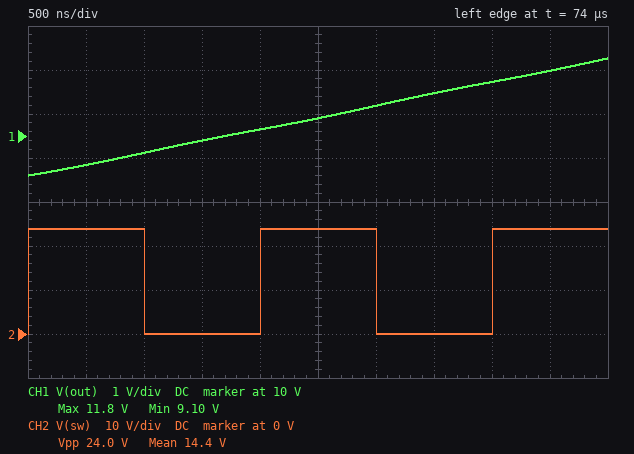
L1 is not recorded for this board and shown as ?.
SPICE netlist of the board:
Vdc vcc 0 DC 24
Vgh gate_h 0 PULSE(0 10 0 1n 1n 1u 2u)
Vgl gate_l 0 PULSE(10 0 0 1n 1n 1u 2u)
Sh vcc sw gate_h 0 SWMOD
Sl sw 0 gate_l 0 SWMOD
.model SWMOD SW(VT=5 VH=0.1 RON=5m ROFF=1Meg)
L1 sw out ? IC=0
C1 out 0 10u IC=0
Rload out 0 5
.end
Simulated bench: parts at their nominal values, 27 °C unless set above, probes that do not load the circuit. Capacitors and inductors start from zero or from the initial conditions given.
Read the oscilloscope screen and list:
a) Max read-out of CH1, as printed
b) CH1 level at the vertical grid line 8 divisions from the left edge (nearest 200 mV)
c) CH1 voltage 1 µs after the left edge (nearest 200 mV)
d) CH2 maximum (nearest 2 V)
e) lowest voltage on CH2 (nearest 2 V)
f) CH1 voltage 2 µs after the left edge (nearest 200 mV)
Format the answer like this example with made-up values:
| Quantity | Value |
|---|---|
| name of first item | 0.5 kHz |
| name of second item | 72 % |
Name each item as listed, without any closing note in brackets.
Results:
| Quantity | Value |
|---|---|
| Max read-out of CH1, as printed | 11.8 V |
| CH1 level at the vertical grid line 8 divisions from the left edge | 11.2 V |
| CH1 voltage 1 µs after the left edge | 9.6 V |
| CH2 maximum | 24 V |
| lowest voltage on CH2 | 0 V |
| CH1 voltage 2 µs after the left edge | 10.2 V |
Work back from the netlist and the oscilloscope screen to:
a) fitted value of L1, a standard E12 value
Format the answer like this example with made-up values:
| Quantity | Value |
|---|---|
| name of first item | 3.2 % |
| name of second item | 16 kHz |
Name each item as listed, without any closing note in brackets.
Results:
| Quantity | Value |
|---|---|
| fitted value of L1, a standard E12 value | 10 µH |
